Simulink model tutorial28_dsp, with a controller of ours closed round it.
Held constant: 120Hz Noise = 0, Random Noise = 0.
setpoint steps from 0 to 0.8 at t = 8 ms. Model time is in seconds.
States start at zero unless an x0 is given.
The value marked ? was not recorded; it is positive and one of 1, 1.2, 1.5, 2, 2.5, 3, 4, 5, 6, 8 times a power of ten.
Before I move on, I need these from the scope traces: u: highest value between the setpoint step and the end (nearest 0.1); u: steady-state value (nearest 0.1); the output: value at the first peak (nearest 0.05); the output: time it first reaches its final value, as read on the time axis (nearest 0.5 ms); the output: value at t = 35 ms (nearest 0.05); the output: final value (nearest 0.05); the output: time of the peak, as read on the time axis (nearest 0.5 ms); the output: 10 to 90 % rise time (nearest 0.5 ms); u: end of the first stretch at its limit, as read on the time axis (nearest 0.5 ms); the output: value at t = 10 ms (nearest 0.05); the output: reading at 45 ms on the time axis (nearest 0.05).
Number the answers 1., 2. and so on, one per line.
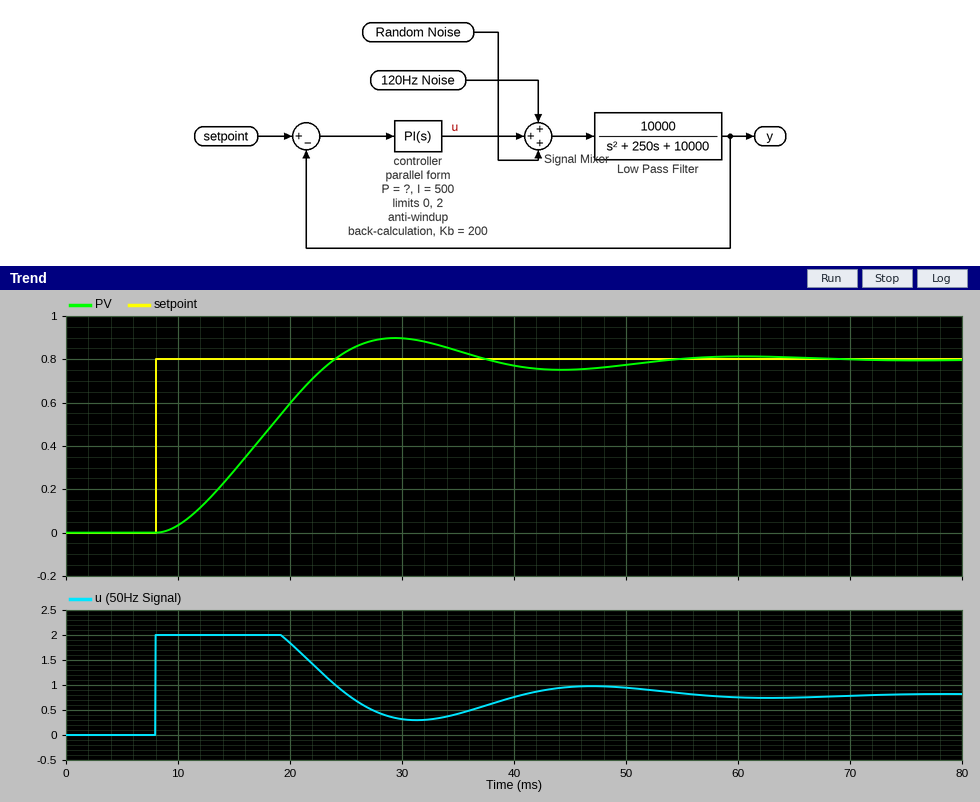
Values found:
1. 2.0
2. 0.8
3. 0.90
4. 24.0 ms
5. 0.85
6. 0.80
7. 29.5 ms
8. 11.0 ms
9. 19.5 ms
10. 0.05
11. 0.75
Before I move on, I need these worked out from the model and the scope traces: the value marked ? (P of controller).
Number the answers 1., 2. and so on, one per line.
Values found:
1. 5
